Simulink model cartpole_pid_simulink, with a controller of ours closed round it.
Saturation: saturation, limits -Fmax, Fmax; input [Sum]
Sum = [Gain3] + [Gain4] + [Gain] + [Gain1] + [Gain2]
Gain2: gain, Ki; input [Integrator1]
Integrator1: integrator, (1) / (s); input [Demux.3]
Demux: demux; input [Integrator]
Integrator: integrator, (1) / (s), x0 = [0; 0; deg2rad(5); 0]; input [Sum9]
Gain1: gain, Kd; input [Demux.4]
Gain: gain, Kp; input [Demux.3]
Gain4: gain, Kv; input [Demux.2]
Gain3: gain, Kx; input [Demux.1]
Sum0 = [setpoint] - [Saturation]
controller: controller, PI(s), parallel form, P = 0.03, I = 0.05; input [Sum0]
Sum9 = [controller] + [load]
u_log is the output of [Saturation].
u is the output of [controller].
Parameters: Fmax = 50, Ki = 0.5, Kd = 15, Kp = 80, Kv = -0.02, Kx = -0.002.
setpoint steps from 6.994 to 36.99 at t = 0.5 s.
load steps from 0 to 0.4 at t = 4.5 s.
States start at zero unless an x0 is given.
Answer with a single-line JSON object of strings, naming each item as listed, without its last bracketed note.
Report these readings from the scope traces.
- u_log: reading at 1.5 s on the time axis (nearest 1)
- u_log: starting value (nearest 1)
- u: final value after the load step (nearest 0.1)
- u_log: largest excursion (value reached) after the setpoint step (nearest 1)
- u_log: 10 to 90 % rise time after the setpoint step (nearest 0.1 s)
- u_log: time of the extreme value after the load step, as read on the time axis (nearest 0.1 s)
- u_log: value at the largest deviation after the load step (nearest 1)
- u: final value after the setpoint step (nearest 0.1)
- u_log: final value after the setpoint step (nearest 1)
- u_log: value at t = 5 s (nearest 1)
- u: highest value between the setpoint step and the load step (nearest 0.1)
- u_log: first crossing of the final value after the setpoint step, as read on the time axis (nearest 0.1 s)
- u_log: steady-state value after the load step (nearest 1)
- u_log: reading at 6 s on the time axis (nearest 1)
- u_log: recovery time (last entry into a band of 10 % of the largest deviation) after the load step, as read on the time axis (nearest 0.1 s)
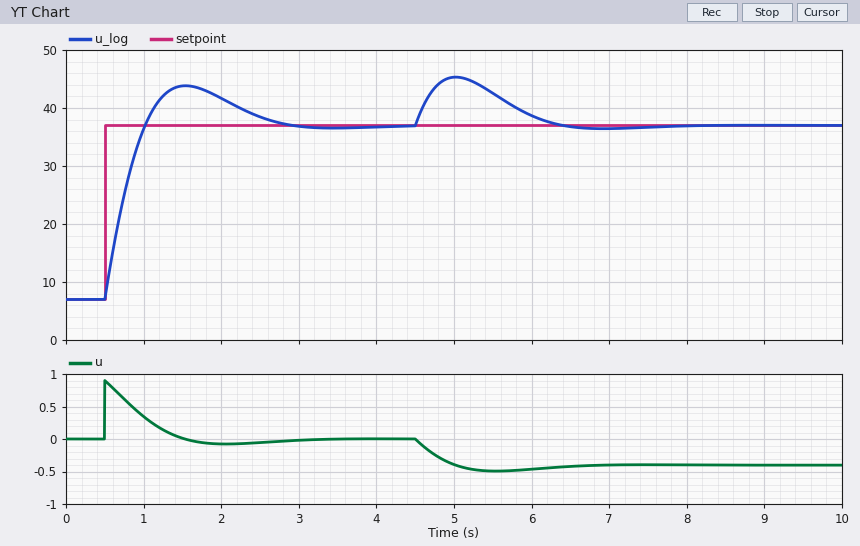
{"u_log: reading at 1.5 s on the time axis": "44", "u_log: starting value": "7", "u: final value after the load step": "-0.4", "u_log: largest excursion (value reached) after the setpoint step": "44", "u_log: 10 to 90 % rise time after the setpoint step": "0.4 s", "u_log: time of the extreme value after the load step, as read on the time axis": "5.0 s", "u_log: value at the largest deviation after the load step": "45", "u: final value after the setpoint step": "0.0", "u_log: final value after the setpoint step": "37", "u_log: value at t = 5 s": "45", "u: highest value between the setpoint step and the load step": "0.9", "u_log: first crossing of the final value after the setpoint step, as read on the time axis": "1.0 s", "u_log: steady-state value after the load step": "37", "u_log: reading at 6 s on the time axis": "39", "u_log: recovery time (last entry into a band of 10 % of the largest deviation) after the load step, as read on the time axis": "6.2 s"}
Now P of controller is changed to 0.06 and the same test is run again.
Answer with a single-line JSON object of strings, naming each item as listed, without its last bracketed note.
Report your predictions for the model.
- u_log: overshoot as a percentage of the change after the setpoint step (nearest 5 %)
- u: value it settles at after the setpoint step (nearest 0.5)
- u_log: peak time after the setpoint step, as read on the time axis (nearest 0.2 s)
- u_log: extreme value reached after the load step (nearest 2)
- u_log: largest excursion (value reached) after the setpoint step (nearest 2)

{"u_log: overshoot as a percentage of the change after the setpoint step": "10 %", "u: value it settles at after the setpoint step": "0.0", "u_log: peak time after the setpoint step, as read on the time axis": "1.4 s", "u_log: extreme value reached after the load step": "42", "u_log: largest excursion (value reached) after the setpoint step": "40"}
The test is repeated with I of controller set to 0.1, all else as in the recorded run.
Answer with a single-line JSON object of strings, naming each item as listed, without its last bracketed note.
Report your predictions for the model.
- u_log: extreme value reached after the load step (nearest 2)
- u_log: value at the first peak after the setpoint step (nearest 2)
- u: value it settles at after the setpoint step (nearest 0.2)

{"u_log: extreme value reached after the load step": "44", "u_log: value at the first peak after the setpoint step": "46", "u: value it settles at after the setpoint step": "0.0"}
